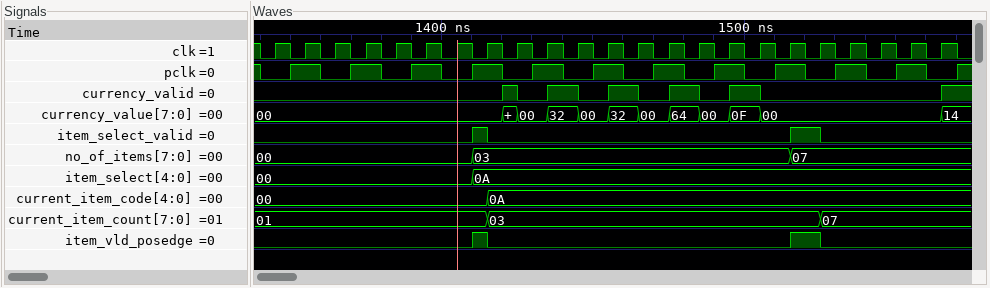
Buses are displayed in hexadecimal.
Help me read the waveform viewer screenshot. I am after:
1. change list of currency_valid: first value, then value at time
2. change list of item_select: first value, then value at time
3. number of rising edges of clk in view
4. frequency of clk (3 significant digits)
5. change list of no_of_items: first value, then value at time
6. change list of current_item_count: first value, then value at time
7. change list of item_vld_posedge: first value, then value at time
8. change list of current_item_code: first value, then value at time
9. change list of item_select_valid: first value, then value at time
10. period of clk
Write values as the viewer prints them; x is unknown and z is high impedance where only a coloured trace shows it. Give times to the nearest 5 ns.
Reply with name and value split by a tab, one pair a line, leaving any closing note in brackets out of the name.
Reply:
change list of currency_valid: first value, then value at time	0, 1 at 1420 ns, 0 at 1425 ns, 1 at 1435 ns, 0 at 1445 ns, 1 at 1455 ns, 0 at 1465 ns, 1 at 1475 ns, 0 at 1485 ns, 1 at 1495 ns, 0 at 1505 ns, 1 at 1565 ns
change list of item_select: first value, then value at time	00, 0A at 1410 ns
number of rising edges of clk in view	23
frequency of clk	100 MHz
change list of no_of_items: first value, then value at time	00, 03 at 1410 ns, 07 at 1515 ns
change list of current_item_count: first value, then value at time	01, 03 at 1415 ns, 07 at 1525 ns
change list of item_vld_posedge: first value, then value at time	0, 1 at 1410 ns, 0 at 1415 ns, 1 at 1515 ns, 0 at 1525 ns
change list of current_item_code: first value, then value at time	00, 0A at 1415 ns
change list of item_select_valid: first value, then value at time	0, 1 at 1410 ns, 0 at 1415 ns, 1 at 1515 ns, 0 at 1525 ns
period of clk	10 ns
